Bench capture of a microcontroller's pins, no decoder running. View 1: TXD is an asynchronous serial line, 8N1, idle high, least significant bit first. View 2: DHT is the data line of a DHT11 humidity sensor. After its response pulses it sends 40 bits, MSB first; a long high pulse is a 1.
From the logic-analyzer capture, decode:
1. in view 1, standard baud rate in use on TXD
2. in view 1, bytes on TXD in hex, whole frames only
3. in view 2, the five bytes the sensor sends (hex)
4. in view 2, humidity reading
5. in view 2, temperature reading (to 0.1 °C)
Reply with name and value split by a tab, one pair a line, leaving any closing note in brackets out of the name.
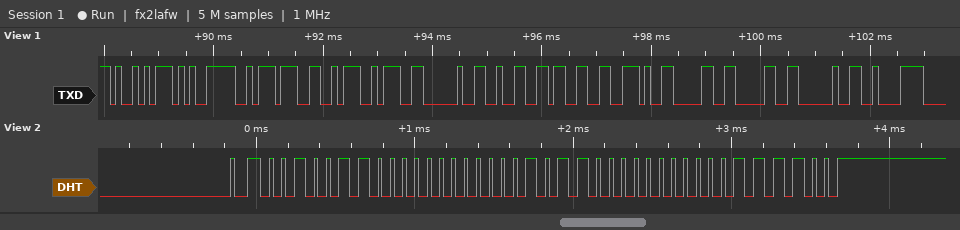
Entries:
in view 1, standard baud rate in use on TXD	9600 baud
in view 1, bytes on TXD in hex, whole frames only	0xA9 0xE5 0xBA 0xA6 0x3A 0x20 0x32 0x33 0x2E 0x30 0x30 0x20 0xC2
in view 2, the five bytes the sensor sends	26 00 16 00 3C
in view 2, humidity reading	38 %
in view 2, temperature reading	22.0 °C
